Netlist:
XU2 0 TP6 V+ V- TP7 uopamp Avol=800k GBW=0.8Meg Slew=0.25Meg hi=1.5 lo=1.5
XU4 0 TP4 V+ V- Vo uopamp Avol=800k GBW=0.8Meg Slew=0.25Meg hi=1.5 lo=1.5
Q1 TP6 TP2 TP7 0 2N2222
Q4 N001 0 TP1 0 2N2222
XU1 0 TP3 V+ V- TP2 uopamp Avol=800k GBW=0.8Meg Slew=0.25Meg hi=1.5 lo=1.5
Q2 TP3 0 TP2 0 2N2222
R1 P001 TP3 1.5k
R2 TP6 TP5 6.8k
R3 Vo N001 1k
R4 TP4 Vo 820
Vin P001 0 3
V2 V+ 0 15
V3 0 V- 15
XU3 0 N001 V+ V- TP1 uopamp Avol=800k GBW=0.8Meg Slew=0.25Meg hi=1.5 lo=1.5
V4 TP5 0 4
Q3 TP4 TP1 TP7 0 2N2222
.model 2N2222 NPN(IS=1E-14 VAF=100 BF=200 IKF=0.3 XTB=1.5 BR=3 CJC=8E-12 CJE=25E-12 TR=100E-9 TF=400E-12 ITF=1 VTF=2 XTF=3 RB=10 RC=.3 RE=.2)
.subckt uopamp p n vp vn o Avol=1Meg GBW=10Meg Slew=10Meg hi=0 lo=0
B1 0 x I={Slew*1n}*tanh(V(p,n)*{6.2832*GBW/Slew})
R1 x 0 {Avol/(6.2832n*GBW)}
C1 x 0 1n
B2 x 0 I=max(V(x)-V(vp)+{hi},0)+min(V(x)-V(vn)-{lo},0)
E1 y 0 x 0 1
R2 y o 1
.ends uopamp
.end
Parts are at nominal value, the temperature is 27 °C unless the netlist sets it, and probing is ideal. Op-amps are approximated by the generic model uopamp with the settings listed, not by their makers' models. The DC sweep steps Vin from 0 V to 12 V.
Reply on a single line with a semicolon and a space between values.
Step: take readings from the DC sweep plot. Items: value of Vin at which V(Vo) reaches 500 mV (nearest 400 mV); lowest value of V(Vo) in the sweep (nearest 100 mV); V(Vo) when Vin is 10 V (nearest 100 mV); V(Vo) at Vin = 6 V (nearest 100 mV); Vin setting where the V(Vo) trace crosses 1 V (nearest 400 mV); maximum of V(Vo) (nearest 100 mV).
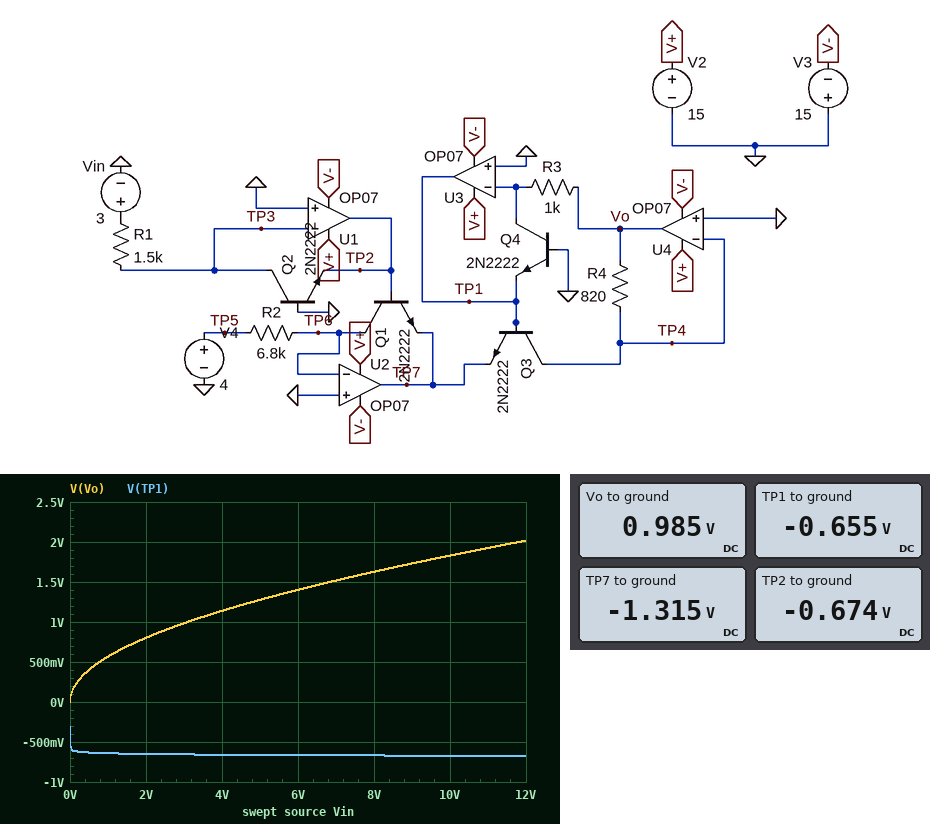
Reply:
800 mV; 0 V; 1.8 V; 1.4 V; 3.2 V; 2.0 V
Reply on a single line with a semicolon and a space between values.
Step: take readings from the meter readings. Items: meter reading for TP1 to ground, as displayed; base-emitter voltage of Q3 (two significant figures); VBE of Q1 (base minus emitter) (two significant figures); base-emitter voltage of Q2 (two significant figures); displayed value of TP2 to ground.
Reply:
-0.655 V; 660 mV; 640 mV; 670 mV; -0.674 V
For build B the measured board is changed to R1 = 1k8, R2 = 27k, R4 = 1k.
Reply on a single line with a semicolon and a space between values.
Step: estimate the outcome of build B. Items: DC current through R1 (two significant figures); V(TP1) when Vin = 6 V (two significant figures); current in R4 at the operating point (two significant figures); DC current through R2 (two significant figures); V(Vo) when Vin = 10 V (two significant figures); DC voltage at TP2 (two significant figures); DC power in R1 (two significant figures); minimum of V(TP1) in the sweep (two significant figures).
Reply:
1.7 mA; -650 mV; 500 µA; 150 µA; 930 mV; -670 mV; 5.0 mW; -660 mV
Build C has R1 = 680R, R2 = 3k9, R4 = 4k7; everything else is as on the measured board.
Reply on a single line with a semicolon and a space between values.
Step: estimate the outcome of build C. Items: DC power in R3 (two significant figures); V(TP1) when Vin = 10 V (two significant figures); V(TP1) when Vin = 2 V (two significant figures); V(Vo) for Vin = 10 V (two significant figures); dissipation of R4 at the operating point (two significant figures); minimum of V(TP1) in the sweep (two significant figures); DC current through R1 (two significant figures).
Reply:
21 mW; -710 mV; -690 mV; 8.7 V; 4.5 mW; -720 mV; 4.4 mA
